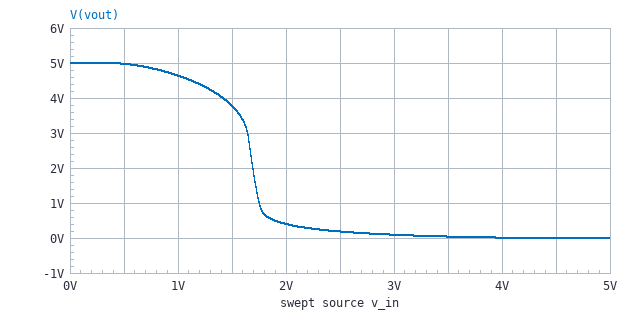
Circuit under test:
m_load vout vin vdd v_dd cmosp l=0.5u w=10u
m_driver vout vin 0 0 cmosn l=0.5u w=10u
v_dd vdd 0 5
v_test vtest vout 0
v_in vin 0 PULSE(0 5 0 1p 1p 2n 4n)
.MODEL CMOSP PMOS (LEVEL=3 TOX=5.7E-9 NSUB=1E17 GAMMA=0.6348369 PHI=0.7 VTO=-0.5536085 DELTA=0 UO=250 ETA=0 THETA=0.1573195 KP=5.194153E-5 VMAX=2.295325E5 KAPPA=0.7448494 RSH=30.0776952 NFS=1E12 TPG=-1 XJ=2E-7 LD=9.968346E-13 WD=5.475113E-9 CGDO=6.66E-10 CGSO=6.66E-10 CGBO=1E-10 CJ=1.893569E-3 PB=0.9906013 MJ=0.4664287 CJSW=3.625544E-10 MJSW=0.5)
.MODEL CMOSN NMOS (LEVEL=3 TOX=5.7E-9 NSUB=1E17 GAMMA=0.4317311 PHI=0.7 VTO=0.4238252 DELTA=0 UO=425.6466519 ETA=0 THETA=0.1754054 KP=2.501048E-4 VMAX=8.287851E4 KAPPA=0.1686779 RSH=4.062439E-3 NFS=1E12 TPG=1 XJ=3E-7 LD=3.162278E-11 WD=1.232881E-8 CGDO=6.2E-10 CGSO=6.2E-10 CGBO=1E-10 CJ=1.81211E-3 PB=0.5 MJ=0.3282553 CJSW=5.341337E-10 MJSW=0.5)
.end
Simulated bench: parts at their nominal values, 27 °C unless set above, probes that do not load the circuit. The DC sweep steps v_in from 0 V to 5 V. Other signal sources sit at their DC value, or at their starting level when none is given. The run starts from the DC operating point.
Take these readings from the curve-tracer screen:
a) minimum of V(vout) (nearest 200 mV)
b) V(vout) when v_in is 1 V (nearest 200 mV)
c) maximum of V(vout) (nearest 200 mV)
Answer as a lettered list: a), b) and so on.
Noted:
a) 0 V
b) 4.6 V
c) 5.0 V
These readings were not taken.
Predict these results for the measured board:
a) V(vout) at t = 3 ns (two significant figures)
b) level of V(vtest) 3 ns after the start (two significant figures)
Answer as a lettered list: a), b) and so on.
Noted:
a) 5.0 V
b) 5.0 V
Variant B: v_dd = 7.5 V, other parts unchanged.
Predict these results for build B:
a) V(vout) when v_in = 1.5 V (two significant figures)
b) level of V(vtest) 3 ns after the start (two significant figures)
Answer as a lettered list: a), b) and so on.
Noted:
a) 6.7 V
b) 7.5 V
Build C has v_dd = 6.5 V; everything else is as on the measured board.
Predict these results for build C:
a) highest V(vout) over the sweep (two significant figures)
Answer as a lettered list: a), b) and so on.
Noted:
a) 6.5 V
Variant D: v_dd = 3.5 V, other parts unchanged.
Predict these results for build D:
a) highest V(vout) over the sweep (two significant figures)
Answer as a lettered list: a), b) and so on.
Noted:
a) 3.5 V
